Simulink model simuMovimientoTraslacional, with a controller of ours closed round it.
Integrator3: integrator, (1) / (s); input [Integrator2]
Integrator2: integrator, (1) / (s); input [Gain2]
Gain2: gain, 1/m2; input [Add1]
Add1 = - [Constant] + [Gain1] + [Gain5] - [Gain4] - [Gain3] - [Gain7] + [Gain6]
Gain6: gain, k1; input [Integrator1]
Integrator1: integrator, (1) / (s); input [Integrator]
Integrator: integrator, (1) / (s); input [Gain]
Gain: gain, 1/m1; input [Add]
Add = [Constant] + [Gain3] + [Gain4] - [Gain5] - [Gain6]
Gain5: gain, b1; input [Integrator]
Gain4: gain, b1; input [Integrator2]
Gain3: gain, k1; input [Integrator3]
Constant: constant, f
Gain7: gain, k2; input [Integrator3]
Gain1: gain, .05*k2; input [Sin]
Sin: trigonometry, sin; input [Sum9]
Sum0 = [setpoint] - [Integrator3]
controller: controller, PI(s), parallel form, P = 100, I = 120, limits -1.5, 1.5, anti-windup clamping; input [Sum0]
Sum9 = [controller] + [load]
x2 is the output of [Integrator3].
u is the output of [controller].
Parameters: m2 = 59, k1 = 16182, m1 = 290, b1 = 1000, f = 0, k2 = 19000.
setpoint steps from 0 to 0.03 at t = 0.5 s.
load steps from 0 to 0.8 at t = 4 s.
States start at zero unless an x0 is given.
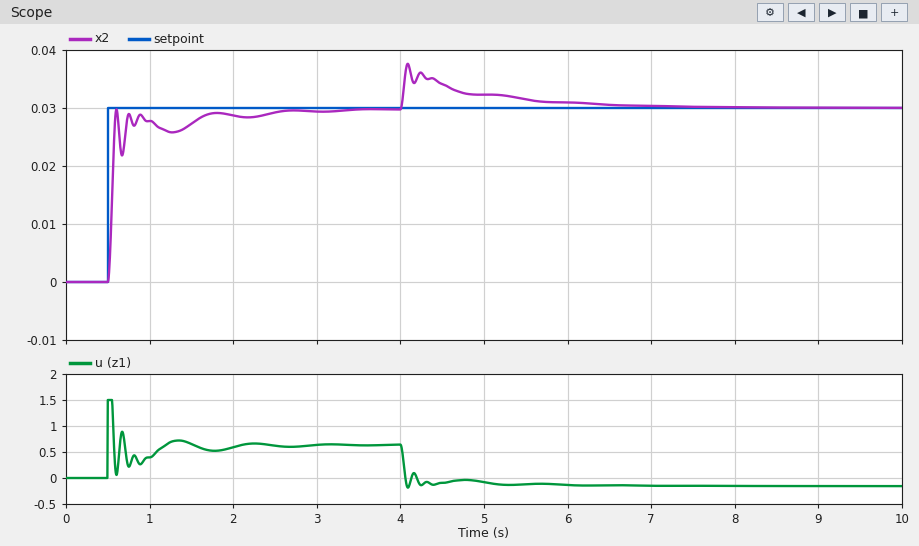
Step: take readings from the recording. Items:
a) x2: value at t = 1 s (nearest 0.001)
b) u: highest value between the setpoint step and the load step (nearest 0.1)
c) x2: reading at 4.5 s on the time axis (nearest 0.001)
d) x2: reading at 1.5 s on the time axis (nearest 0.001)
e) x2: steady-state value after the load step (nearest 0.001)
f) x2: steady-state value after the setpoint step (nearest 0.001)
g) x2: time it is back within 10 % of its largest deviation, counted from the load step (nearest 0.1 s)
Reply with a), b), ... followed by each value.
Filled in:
a) 0.028
b) 1.5
c) 0.034
d) 0.027
e) 0.030
f) 0.030
g) 2.3 s
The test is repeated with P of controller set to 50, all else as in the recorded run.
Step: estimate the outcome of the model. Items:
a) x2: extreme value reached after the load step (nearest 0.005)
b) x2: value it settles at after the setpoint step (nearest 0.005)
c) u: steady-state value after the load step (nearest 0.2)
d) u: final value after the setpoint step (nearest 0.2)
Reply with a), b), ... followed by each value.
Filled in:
a) 0.040
b) 0.030
c) -0.2
d) 0.6
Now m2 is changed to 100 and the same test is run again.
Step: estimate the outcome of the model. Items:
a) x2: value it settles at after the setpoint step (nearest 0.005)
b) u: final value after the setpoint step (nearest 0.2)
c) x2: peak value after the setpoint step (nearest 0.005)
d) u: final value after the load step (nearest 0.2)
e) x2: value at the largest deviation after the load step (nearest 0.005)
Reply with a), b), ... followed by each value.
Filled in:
a) 0.030
b) 0.6
c) 0.030
d) -0.2
e) 0.040
